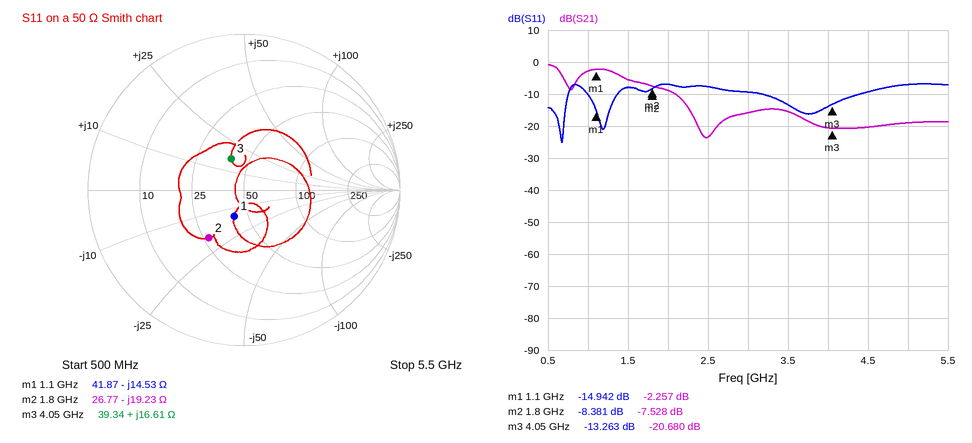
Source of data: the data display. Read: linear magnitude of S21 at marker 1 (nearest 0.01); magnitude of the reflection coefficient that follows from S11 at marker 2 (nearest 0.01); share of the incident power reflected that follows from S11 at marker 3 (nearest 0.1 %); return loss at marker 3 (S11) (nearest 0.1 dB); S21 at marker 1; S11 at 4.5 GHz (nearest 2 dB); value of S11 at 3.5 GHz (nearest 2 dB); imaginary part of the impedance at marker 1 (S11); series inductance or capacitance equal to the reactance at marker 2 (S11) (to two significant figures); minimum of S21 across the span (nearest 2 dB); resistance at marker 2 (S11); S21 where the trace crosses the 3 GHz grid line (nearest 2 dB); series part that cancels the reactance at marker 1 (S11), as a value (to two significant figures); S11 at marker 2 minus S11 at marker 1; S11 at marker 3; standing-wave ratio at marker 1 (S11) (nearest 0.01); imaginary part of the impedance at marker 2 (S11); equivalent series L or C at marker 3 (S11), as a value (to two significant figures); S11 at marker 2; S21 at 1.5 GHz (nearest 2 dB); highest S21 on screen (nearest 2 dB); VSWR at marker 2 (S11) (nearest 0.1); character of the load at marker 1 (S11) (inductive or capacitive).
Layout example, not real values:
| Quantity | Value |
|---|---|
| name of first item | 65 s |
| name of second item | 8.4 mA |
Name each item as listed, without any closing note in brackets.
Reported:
| Quantity | Value |
|---|---|
| linear magnitude of S21 at marker 1 | 0.77 |
| magnitude of the reflection coefficient that follows from S11 at marker 2 | 0.38 |
| share of the incident power reflected that follows from S11 at marker 3 | 4.7 % |
| return loss at marker 3 (S11) | 13.3 dB |
| S21 at marker 1 | -2.257 dB |
| S11 at 4.5 GHz | -10 dB |
| value of S11 at 3.5 GHz | -14 dB |
| imaginary part of the impedance at marker 1 | -14.53 Ω |
| series inductance or capacitance equal to the reactance at marker 2 (S11) | 4.6 pF |
| minimum of S21 across the span | -24 dB |
| resistance at marker 2 | 26.77 Ω |
| S21 where the trace crosses the 3 GHz grid line | -16 dB |
| series part that cancels the reactance at marker 1 (S11), as a value | 2.1 nH |
| S11 at marker 2 minus S11 at marker 1 | 6.561 dB |
| S11 at marker 3 | -13.263 dB |
| standing-wave ratio at marker 1 (S11) | 1.44 |
| imaginary part of the impedance at marker 2 | -19.23 Ω |
| equivalent series L or C at marker 3 (S11), as a value | 650 pH |
| S11 at marker 2 | -8.381 dB |
| S21 at 1.5 GHz | -6 dB |
| highest S21 on screen | 0 dB |
| VSWR at marker 2 (S11) | 2.2 |
| character of the load at marker 1 (S11) | capacitive |
